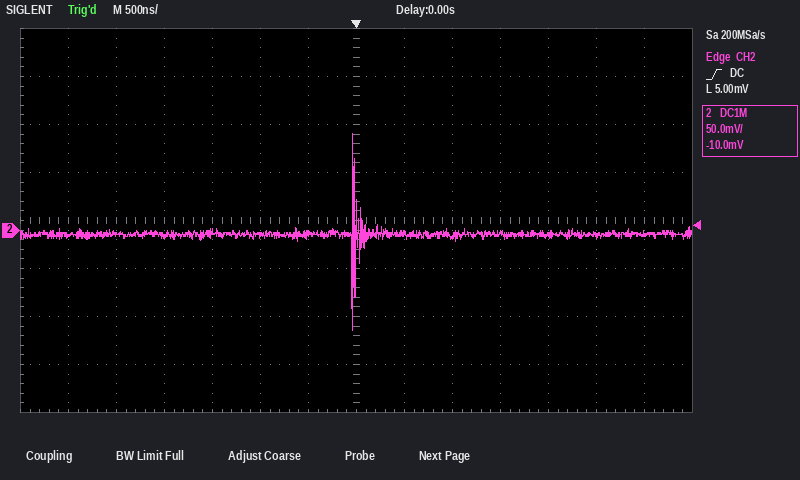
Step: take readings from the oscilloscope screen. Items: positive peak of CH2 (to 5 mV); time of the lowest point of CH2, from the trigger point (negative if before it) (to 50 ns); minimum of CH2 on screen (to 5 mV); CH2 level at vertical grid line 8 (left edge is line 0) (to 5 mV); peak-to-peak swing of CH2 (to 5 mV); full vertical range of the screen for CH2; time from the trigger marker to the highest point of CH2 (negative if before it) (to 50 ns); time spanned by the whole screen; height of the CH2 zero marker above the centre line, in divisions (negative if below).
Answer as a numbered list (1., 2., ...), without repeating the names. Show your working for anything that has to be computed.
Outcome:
1. 100 mV
2. -50 ns
3. -105 mV
4. -5 mV
5. 100 mV − (-105 mV) = 205 mV
6. 400 mV
7. -50 ns
8. 7 µs
9. -0.2 div
